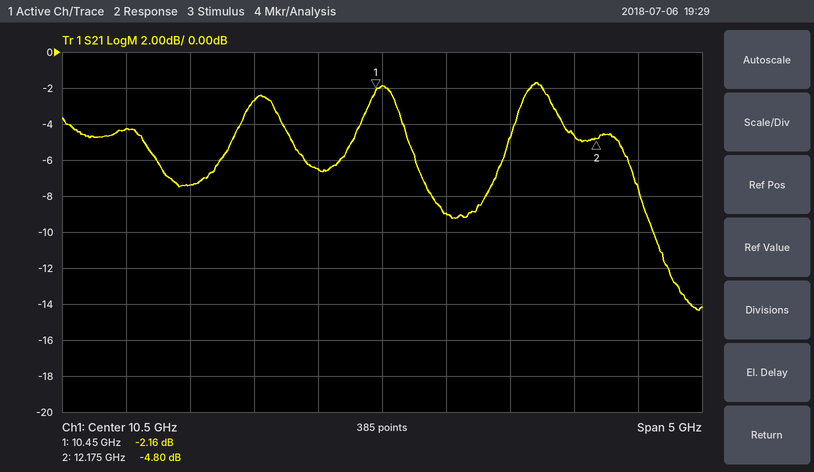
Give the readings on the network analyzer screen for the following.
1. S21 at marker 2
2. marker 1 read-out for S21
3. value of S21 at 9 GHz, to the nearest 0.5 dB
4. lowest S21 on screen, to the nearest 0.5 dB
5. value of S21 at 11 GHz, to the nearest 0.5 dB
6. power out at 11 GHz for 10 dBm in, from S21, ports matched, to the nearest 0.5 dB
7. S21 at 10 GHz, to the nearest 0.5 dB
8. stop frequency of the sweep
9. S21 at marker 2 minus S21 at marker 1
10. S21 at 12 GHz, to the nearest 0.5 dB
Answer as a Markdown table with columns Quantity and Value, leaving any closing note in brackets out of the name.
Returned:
| Quantity | Value |
|---|---|
| S21 at marker 2 | -4.80 dB |
| marker 1 read-out for S21 | -2.16 dB |
| value of S21 at 9 GHz, to the nearest 0.5 dB | -7.5 dB |
| lowest S21 on screen, to the nearest 0.5 dB | -14.5 dB |
| value of S21 at 11 GHz, to the nearest 0.5 dB | -9.0 dB |
| power out at 11 GHz for 10 dBm in, from S21, ports matched, to the nearest 0.5 dB | 1.0 dBm |
| S21 at 10 GHz, to the nearest 0.5 dB | -6.5 dB |
| stop frequency of the sweep | 13 GHz |
| S21 at marker 2 minus S21 at marker 1 | -2.64 dB |
| S21 at 12 GHz, to the nearest 0.5 dB | -4.5 dB |
